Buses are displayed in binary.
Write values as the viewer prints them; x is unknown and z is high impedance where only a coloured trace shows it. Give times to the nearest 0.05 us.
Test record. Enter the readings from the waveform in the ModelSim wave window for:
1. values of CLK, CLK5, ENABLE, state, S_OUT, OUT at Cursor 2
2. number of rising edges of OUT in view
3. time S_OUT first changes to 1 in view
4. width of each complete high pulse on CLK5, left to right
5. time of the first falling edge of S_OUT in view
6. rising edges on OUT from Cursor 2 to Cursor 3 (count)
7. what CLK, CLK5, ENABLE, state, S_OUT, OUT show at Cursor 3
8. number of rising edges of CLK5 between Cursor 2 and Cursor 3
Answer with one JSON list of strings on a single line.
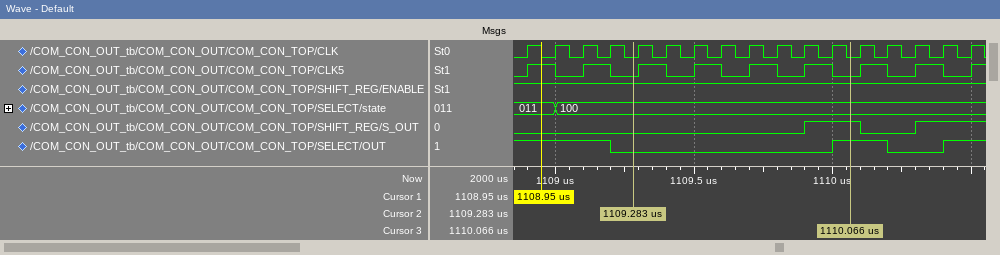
["CLK=0, CLK5=0, ENABLE=1, state=100, S_OUT=0, OUT=0", "2", "1109.9 us", "0.1 us, 0.1 us, 0.1 us, 0.1 us, 0.1 us, 0.1 us, 0.1 us, 0.1 us", "1110.1 us", "1", "CLK=0, CLK5=0, ENABLE=1, state=100, S_OUT=1, OUT=1", "4"]
